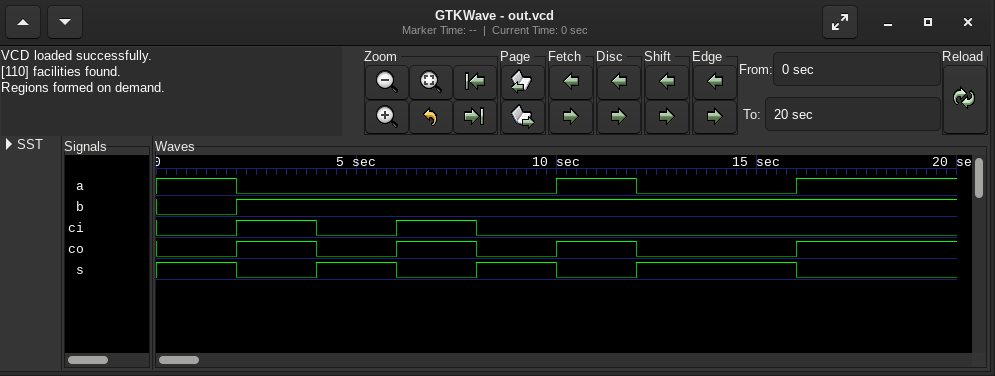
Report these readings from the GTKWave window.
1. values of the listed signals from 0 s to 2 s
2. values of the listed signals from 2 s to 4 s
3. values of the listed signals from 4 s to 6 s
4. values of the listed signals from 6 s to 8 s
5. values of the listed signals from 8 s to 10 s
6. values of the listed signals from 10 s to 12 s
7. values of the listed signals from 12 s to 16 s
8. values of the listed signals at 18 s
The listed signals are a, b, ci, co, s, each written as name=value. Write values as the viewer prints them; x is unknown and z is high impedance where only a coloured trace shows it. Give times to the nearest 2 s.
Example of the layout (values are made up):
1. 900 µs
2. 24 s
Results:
1. a=1, b=0, ci=0, co=0, s=1
2. a=0, b=1, ci=1, co=1, s=0
3. a=0, b=1, ci=0, co=0, s=1
4. a=0, b=1, ci=1, co=1, s=0
5. a=0, b=1, ci=0, co=0, s=1
6. a=1, b=1, ci=0, co=1, s=0
7. a=0, b=1, ci=0, co=0, s=1
8. a=1, b=1, ci=0, co=1, s=0
